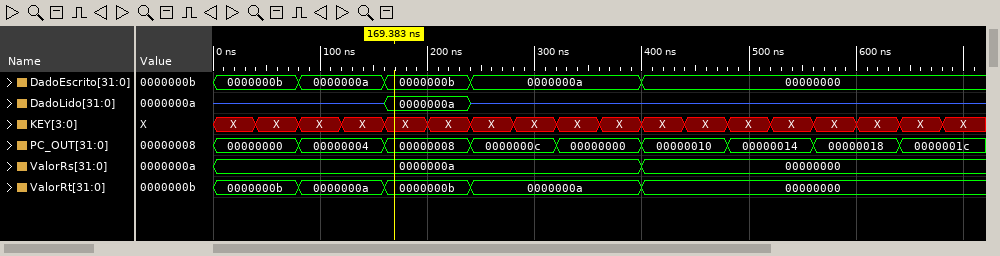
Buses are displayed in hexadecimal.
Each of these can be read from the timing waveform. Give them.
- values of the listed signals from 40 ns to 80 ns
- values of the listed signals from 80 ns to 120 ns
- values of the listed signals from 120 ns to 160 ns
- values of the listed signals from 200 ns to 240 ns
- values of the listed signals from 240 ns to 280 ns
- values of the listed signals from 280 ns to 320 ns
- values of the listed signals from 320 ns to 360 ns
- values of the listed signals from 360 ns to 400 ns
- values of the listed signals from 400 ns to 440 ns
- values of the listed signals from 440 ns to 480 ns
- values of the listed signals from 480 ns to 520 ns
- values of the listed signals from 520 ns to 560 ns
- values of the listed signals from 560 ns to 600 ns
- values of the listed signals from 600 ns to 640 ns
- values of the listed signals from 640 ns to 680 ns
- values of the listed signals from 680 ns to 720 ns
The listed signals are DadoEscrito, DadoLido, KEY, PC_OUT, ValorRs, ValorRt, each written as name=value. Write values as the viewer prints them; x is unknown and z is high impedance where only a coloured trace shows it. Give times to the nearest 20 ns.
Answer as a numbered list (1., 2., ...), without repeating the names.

1. DadoEscrito=0000000b, DadoLido=z, KEY=X, PC_OUT=00000000, ValorRs=0000000a, ValorRt=0000000b
2. DadoEscrito=0000000a, DadoLido=z, KEY=X, PC_OUT=00000004, ValorRs=0000000a, ValorRt=0000000a
3. DadoEscrito=0000000a, DadoLido=z, KEY=X, PC_OUT=00000004, ValorRs=0000000a, ValorRt=0000000a
4. DadoEscrito=0000000b, DadoLido=0000000a, KEY=X, PC_OUT=00000008, ValorRs=0000000a, ValorRt=0000000b
5. DadoEscrito=0000000a, DadoLido=z, KEY=X, PC_OUT=0000000c, ValorRs=0000000a, ValorRt=0000000a
6. DadoEscrito=0000000a, DadoLido=z, KEY=X, PC_OUT=0000000c, ValorRs=0000000a, ValorRt=0000000a
7. DadoEscrito=0000000a, DadoLido=z, KEY=X, PC_OUT=00000000, ValorRs=0000000a, ValorRt=0000000a
8. DadoEscrito=0000000a, DadoLido=z, KEY=X, PC_OUT=00000000, ValorRs=0000000a, ValorRt=0000000a
9. DadoEscrito=00000000, DadoLido=z, KEY=X, PC_OUT=00000010, ValorRs=00000000, ValorRt=00000000
10. DadoEscrito=00000000, DadoLido=z, KEY=X, PC_OUT=00000010, ValorRs=00000000, ValorRt=00000000
11. DadoEscrito=00000000, DadoLido=z, KEY=X, PC_OUT=00000014, ValorRs=00000000, ValorRt=00000000
12. DadoEscrito=00000000, DadoLido=z, KEY=X, PC_OUT=00000014, ValorRs=00000000, ValorRt=00000000
13. DadoEscrito=00000000, DadoLido=z, KEY=X, PC_OUT=00000018, ValorRs=00000000, ValorRt=00000000
14. DadoEscrito=00000000, DadoLido=z, KEY=X, PC_OUT=00000018, ValorRs=00000000, ValorRt=00000000
15. DadoEscrito=00000000, DadoLido=z, KEY=X, PC_OUT=0000001c, ValorRs=00000000, ValorRt=00000000
16. DadoEscrito=00000000, DadoLido=z, KEY=X, PC_OUT=0000001c, ValorRs=00000000, ValorRt=00000000
